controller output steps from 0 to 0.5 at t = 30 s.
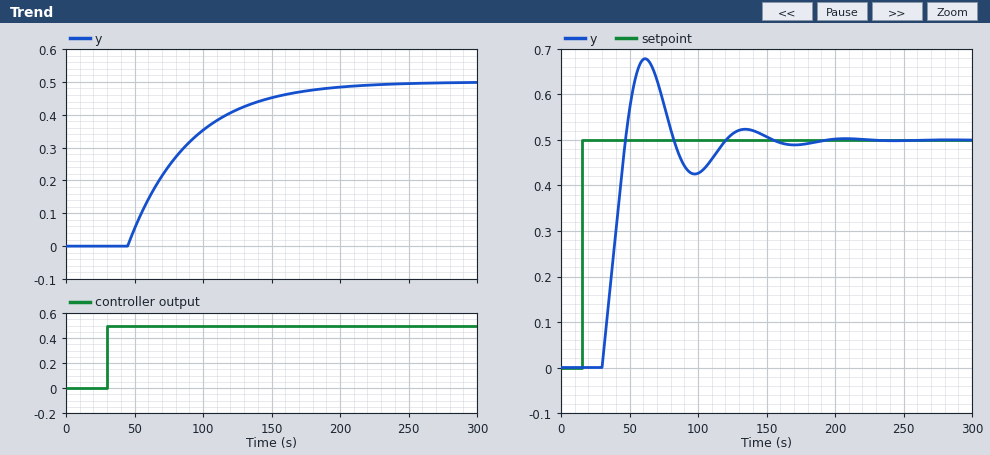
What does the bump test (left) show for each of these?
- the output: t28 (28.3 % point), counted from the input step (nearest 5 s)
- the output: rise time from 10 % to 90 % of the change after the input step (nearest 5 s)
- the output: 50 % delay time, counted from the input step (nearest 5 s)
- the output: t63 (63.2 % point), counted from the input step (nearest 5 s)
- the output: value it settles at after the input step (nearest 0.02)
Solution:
30 s
100 s
45 s
60 s
0.50
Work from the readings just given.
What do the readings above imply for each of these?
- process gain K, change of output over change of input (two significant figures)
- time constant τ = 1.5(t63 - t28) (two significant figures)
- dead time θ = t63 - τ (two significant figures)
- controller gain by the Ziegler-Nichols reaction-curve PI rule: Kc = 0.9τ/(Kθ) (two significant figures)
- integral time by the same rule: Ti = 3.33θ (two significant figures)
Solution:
1.0
45 s
15 s
2.7
50 s
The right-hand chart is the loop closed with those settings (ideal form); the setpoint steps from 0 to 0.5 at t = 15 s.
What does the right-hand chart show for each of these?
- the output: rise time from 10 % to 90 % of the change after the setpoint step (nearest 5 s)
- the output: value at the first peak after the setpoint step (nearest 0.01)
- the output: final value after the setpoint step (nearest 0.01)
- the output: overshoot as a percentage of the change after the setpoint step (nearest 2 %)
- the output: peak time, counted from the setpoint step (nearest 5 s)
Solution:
15 s
0.68
0.50
36 %
45 s
